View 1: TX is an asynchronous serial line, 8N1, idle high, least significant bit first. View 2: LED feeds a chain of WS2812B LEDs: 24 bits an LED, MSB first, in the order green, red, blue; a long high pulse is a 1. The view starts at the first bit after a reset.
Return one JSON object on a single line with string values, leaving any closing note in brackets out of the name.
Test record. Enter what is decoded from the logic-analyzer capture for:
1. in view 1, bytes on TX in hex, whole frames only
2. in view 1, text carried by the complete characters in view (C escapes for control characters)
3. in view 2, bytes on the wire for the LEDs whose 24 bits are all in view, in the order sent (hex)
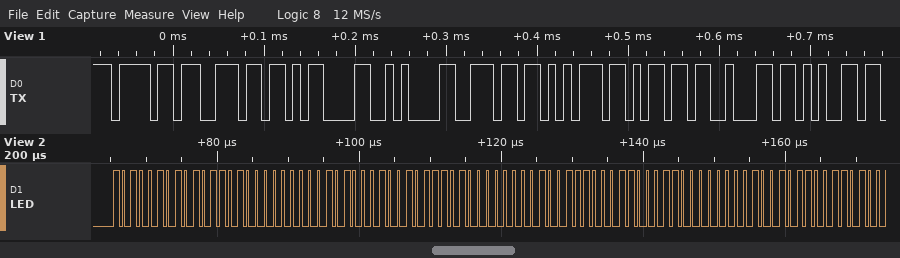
{"in view 1, bytes on TX in hex, whole frames only": "6F 6E 0D 0A 6E 75 6D 62 65", "in view 1, text carried by the complete characters in view": "\"on\\r\\nnumbe\"", "in view 2, bytes on the wire for the LEDs whose 24 bits are all in view, in the order sent": "A5 5A 00 A2 5D 00 9C 63 00"}
